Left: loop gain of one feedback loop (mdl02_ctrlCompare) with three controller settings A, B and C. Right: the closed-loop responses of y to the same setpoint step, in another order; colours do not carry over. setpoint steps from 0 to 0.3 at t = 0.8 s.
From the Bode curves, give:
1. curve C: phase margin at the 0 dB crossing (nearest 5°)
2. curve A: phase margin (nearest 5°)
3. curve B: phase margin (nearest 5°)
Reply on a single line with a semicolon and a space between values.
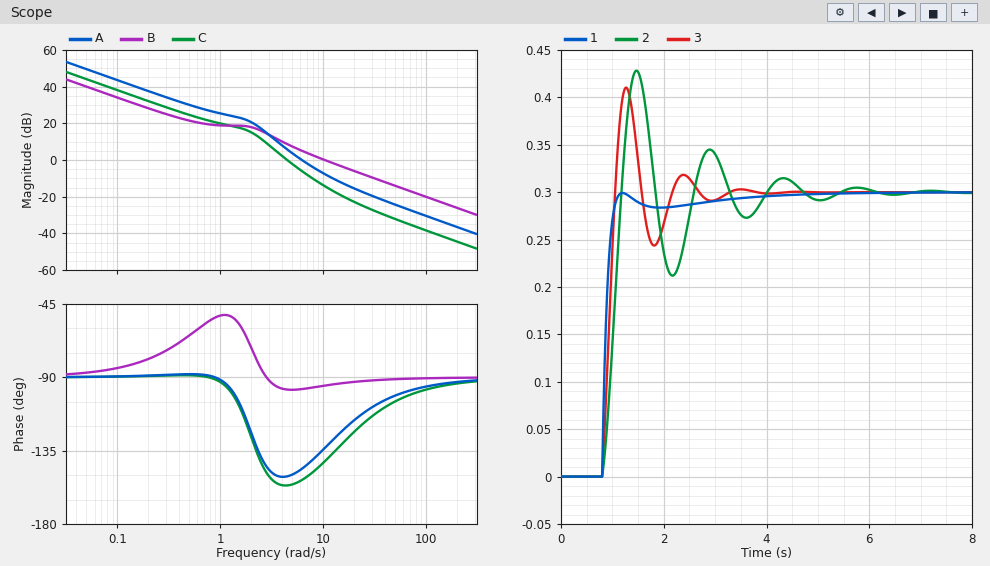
25°; 35°; 85°
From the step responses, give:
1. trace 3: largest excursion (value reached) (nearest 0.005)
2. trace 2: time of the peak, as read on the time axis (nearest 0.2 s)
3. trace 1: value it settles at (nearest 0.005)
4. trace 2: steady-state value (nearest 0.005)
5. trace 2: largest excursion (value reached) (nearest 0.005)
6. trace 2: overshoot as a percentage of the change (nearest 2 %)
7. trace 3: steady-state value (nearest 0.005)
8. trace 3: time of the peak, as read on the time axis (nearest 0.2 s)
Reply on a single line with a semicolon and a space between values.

0.410; 1.4 s; 0.300; 0.300; 0.430; 42 %; 0.300; 1.2 s
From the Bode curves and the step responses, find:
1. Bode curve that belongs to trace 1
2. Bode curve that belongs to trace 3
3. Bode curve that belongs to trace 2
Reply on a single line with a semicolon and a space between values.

B; A; C
